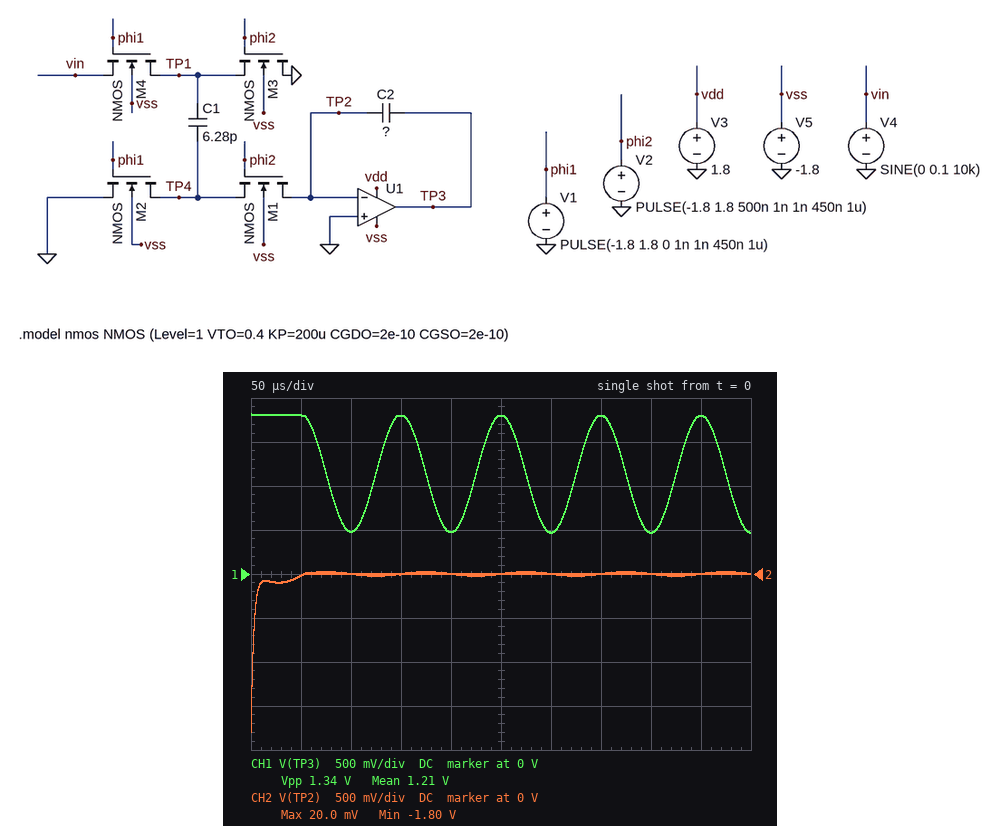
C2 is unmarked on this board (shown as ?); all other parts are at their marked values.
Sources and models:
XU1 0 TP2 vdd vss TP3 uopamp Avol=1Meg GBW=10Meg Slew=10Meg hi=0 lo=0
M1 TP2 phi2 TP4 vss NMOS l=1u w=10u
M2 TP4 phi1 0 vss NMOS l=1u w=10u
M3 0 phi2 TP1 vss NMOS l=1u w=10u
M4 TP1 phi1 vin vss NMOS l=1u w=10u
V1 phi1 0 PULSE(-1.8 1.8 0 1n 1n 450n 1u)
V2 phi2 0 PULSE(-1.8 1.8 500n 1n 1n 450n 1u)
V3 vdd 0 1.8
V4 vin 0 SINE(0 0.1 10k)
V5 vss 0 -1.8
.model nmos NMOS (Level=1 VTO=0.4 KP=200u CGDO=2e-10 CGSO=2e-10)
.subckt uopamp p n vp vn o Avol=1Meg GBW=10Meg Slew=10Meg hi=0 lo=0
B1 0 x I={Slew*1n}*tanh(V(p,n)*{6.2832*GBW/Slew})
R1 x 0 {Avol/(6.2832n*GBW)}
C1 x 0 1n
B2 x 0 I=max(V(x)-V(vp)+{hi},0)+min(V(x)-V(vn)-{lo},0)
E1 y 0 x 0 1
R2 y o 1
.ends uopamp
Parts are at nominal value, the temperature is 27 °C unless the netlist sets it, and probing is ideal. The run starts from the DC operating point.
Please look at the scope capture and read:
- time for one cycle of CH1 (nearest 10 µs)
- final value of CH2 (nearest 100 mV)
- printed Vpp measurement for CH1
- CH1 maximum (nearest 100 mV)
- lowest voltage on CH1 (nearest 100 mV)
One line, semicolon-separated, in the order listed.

100 µs; 0 V; 1.34 V; 1.8 V; 500 mV
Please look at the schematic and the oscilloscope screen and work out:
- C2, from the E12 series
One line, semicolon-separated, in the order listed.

15 pF
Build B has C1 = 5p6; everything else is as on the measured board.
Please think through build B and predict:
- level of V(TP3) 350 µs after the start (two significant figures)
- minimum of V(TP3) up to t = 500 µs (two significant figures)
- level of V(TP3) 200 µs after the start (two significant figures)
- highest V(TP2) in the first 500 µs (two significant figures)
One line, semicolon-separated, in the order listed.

1.8 V; 610 mV; 620 mV; 20 mV
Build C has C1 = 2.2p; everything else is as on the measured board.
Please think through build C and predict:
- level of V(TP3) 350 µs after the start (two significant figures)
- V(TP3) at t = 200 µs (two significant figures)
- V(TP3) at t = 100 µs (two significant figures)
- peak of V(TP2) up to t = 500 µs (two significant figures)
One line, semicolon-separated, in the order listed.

1.8 V; 1.3 V; 1.4 V; 11 mV
